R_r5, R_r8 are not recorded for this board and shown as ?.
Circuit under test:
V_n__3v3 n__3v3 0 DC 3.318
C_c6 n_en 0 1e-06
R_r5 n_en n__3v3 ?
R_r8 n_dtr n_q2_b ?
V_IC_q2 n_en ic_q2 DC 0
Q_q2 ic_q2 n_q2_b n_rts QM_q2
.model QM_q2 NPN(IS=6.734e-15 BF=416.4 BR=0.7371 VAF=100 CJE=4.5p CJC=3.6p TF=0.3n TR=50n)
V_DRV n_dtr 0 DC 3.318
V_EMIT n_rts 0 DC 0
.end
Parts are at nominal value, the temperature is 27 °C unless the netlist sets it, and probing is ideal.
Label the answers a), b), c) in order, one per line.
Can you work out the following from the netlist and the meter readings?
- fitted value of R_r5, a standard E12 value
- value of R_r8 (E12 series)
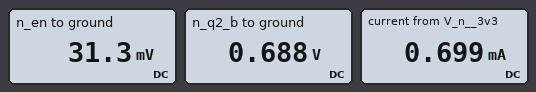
a) 4.7 kΩ
b) 2.7 kΩ
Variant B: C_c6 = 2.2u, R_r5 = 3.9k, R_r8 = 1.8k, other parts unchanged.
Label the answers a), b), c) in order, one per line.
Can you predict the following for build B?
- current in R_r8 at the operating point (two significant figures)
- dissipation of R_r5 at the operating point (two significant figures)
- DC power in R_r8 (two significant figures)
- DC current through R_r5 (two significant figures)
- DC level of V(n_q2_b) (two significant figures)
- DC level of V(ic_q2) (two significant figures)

a) 1.5 mA
b) 2.8 mW
c) 3.8 mW
d) 840 µA
e) 700 mV
f) 30 mV
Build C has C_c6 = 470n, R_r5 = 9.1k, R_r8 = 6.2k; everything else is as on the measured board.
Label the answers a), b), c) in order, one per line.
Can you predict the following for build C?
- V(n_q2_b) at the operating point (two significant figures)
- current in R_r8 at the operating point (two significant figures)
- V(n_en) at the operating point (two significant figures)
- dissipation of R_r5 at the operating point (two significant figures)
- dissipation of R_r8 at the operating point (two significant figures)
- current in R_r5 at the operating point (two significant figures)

a) 670 mV
b) 430 µA
c) 33 mV
d) 1.2 mW
e) 1.1 mW
f) 360 µA
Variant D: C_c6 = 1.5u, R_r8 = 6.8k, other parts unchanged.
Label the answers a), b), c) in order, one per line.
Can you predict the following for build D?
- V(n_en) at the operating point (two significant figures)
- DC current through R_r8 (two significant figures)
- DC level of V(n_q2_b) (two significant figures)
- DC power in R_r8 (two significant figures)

a) 41 mV
b) 390 µA
c) 670 mV
d) 1.0 mW
